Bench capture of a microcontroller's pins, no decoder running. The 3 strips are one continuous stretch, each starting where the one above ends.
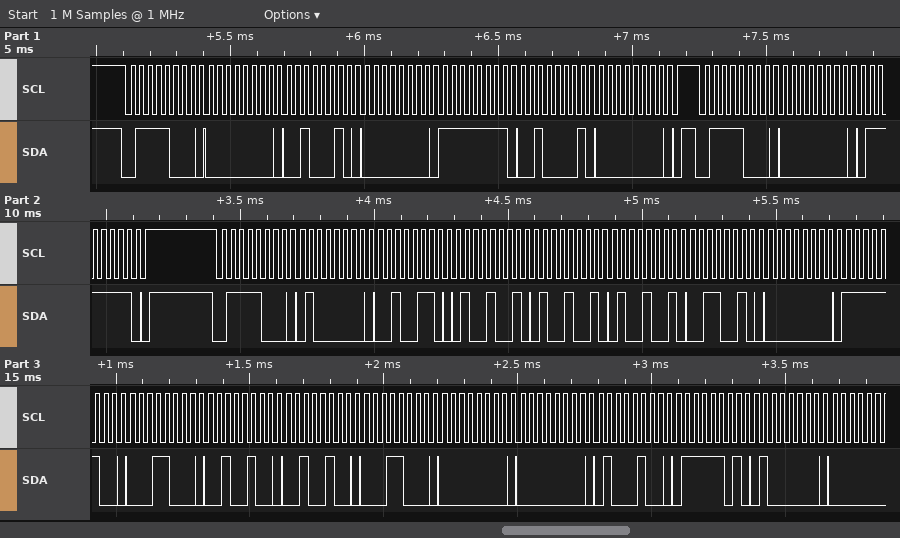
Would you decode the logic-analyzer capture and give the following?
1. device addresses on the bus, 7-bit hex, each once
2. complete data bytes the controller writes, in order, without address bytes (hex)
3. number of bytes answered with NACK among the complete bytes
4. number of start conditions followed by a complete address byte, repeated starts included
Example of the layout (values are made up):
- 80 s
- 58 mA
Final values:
- 0x3C
- 00 22 00 FF 21 00 00 7F 40 26 49 49 49 32 00 FC 18 24 24 18 00 00 44 7D 40
- 0
- 3
